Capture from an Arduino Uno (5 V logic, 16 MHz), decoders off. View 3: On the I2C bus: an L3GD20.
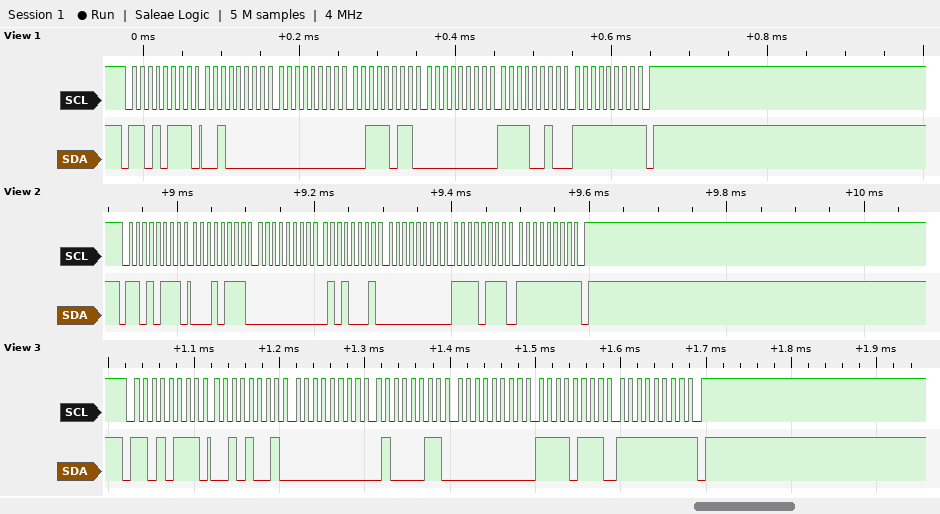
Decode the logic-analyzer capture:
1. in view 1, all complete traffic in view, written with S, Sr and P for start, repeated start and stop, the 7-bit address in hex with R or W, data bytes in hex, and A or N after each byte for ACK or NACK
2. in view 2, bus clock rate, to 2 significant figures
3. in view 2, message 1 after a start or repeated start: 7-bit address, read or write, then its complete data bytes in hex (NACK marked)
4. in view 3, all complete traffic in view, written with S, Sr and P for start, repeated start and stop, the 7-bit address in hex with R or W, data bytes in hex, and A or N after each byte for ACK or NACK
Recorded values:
S 6BR A 20 A 00 A 3B A 00 A F2 A FF N P
100 kHz
0x6B read: 17 00 51 00 F7 FF NACK
S 6BR A 29 A 00 A 43 A 00 A F7 A FF N P
